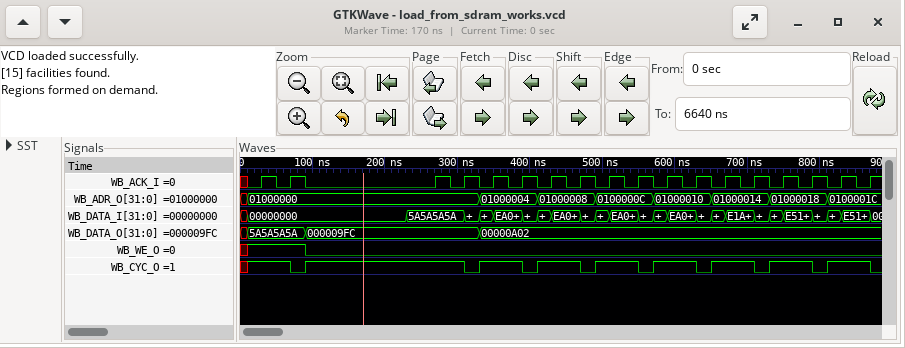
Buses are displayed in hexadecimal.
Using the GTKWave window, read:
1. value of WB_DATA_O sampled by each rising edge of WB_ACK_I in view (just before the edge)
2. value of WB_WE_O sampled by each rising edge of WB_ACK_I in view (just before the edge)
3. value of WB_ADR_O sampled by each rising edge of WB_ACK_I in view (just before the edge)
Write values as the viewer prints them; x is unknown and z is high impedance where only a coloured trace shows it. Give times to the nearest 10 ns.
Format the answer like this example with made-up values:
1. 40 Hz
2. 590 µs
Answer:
1. 5A5A5A5A, 5A5A5A5A, 000009FC, 000009FC, 00000A02, 00000A02, 00000A02, 00000A02, 00000A02, 00000A02, 00000A02, 00000A02, 00000A02, 00000A02, 00000A02, 00000A02, 00000A02, 00000A02
2. 1 1 0 0 0 0 0 0 0 0 0 0 0 0 0 0 0 0
3. 01000000, 01000000, 01000000, 01000000, 01000004, 01000004, 01000008, 01000008, 0100000C, 0100000C, 01000010, 01000010, 01000014, 01000014, 01000018, 01000018, 0100001C, 0100001C
